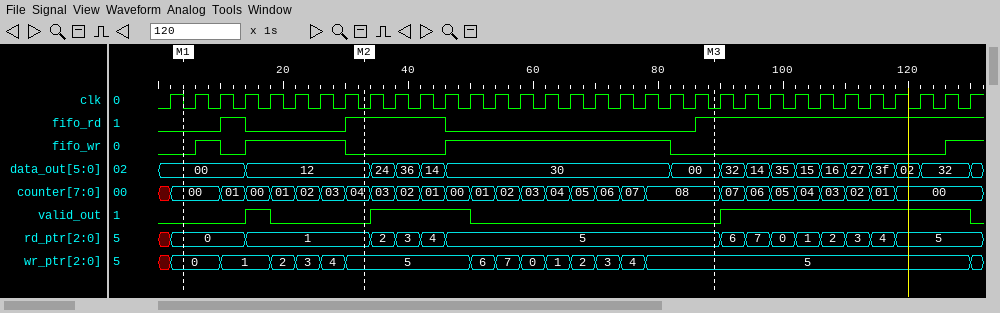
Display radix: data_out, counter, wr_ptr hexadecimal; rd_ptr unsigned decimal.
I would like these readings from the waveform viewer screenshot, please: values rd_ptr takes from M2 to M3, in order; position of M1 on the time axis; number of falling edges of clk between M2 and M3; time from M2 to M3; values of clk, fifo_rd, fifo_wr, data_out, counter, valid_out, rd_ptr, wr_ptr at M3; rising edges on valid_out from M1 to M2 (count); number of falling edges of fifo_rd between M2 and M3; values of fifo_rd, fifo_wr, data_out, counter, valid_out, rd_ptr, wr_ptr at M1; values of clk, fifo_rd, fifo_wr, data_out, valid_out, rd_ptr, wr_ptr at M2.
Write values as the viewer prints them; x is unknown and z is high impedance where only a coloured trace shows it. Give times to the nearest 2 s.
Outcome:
1, 2, 3, 4, 5
4 s
14
56 s
clk=0, fifo_rd=1, fifo_wr=0, data_out=00, counter=08, valid_out=0, rd_ptr=5, wr_ptr=5
1
1
fifo_rd=0, fifo_wr=0, data_out=00, counter=00, valid_out=0, rd_ptr=0, wr_ptr=0
clk=0, fifo_rd=1, fifo_wr=0, data_out=12, valid_out=0, rd_ptr=1, wr_ptr=5
